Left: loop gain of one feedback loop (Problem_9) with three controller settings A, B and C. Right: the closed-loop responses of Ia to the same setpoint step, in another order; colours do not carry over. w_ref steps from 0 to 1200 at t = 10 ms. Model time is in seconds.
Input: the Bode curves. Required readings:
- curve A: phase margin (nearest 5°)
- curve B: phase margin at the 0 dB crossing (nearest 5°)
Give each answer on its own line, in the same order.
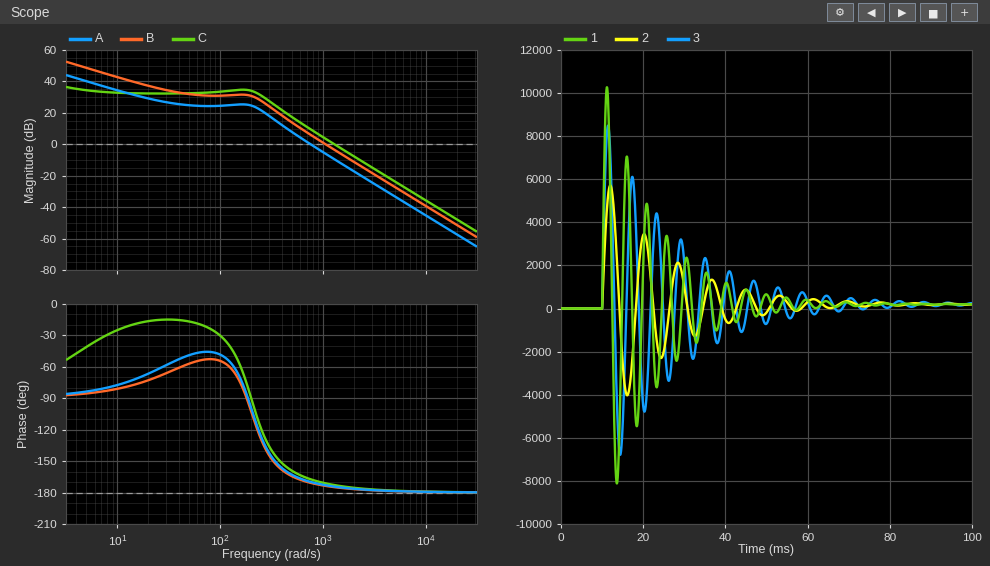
10°
5°
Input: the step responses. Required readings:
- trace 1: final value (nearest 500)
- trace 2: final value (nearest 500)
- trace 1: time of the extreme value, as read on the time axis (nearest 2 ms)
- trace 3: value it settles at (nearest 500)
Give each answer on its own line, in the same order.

0
0
12 ms
0
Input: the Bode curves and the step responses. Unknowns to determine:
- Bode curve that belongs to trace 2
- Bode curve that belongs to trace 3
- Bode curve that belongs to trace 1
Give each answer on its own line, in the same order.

A
B
C
